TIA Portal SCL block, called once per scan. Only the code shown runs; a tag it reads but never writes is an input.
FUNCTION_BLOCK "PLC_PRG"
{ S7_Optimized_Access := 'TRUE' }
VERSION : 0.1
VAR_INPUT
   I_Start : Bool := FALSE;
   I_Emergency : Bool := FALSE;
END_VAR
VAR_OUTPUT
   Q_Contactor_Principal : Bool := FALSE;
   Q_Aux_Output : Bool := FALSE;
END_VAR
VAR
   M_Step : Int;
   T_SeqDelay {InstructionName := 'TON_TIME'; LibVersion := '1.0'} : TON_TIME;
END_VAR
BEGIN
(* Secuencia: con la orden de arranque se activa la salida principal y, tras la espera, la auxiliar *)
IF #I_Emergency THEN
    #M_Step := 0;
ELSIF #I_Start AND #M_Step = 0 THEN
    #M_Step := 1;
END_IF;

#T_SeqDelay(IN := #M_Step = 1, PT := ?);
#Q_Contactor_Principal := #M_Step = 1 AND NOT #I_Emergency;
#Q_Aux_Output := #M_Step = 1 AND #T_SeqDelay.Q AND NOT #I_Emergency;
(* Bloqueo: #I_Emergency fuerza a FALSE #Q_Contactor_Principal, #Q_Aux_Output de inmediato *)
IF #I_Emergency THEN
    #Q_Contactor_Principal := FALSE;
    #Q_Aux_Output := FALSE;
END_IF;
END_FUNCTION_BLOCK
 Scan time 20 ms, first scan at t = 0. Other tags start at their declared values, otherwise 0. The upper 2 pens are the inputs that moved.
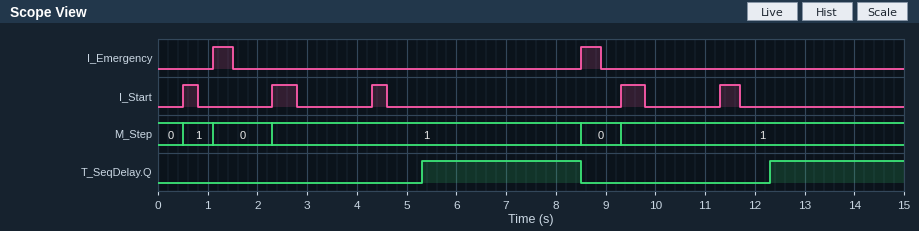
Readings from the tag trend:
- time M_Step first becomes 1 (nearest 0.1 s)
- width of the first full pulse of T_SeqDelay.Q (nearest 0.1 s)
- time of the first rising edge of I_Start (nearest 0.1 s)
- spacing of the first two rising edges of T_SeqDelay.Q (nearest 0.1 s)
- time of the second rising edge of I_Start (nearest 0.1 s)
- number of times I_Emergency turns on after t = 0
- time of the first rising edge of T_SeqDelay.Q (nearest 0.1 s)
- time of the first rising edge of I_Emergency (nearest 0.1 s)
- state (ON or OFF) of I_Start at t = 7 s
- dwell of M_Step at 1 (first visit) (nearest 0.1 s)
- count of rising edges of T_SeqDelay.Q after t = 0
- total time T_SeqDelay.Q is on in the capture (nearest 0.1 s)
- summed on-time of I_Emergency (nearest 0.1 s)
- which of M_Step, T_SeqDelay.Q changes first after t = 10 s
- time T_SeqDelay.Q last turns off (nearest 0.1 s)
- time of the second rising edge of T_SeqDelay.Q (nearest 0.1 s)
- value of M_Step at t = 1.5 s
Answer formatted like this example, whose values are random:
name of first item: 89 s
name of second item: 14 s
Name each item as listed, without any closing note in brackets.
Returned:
time M_Step first becomes 1: 0.5 s
width of the first full pulse of T_SeqDelay.Q: 3.2 s
time of the first rising edge of I_Start: 0.5 s
spacing of the first two rising edges of T_SeqDelay.Q: 7.0 s
time of the second rising edge of I_Start: 2.3 s
number of times I_Emergency turns on after t = 0: 2
time of the first rising edge of T_SeqDelay.Q: 5.3 s
time of the first rising edge of I_Emergency: 1.1 s
state (ON or OFF) of I_Start at t = 7 s: OFF
dwell of M_Step at 1 (first visit): 0.6 s
count of rising edges of T_SeqDelay.Q after t = 0: 2
total time T_SeqDelay.Q is on in the capture: 5.9 s
summed on-time of I_Emergency: 0.8 s
which of M_Step, T_SeqDelay.Q changes first after t = 10 s: T_SeqDelay.Q
time T_SeqDelay.Q last turns off: 8.5 s
time of the second rising edge of T_SeqDelay.Q: 12.3 s
value of M_Step at t = 1.5 s: 0
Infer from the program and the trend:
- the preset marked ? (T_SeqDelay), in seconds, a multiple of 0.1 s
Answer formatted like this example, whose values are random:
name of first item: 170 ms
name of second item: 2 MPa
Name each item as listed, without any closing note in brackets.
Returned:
the preset marked ? (T_SeqDelay), in seconds, a multiple of 0.1 s: 3.0 s
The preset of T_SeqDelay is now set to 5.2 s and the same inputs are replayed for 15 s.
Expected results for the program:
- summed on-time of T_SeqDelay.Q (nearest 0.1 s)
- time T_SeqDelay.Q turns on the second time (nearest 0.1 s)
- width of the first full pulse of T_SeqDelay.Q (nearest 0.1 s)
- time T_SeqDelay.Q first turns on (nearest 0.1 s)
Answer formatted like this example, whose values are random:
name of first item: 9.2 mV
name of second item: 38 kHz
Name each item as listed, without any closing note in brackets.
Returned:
summed on-time of T_SeqDelay.Q: 1.5 s
time T_SeqDelay.Q turns on the second time: 14.5 s
width of the first full pulse of T_SeqDelay.Q: 1.0 s
time T_SeqDelay.Q first turns on: 7.5 s
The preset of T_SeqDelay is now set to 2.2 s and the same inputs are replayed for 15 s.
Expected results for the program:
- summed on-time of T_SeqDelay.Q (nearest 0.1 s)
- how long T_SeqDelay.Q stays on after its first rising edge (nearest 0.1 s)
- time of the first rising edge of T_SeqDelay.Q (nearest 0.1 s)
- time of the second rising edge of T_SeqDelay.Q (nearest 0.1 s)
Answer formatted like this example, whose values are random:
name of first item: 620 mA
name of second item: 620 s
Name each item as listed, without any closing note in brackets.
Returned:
summed on-time of T_SeqDelay.Q: 7.5 s
how long T_SeqDelay.Q stays on after its first rising edge: 4.0 s
time of the first rising edge of T_SeqDelay.Q: 4.5 s
time of the second rising edge of T_SeqDelay.Q: 11.5 s
